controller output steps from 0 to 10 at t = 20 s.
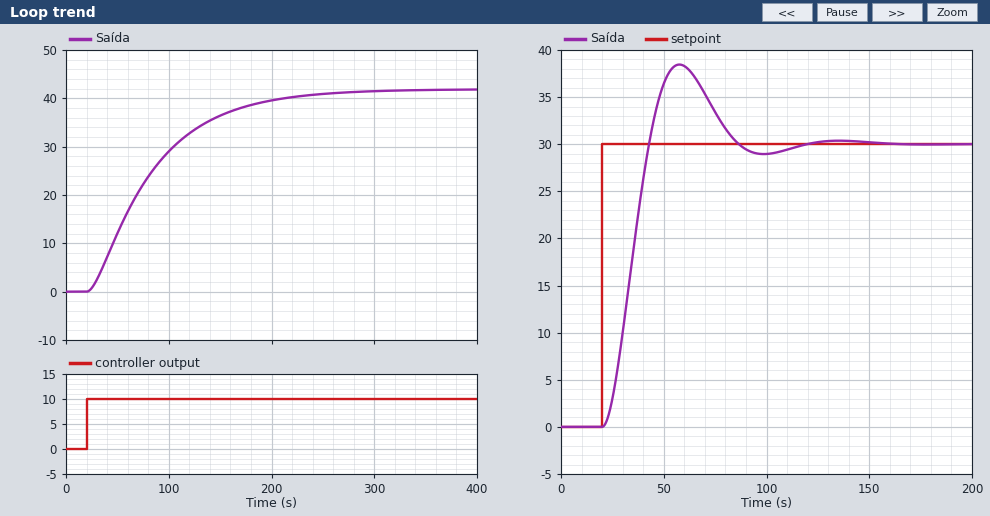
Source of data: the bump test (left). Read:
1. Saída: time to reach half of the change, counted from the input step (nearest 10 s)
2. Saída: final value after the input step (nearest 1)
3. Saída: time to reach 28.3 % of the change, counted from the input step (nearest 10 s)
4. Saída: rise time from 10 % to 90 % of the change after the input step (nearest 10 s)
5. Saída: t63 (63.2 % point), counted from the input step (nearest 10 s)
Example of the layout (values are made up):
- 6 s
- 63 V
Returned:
- 50 s
- 42
- 30 s
- 130 s
- 70 s
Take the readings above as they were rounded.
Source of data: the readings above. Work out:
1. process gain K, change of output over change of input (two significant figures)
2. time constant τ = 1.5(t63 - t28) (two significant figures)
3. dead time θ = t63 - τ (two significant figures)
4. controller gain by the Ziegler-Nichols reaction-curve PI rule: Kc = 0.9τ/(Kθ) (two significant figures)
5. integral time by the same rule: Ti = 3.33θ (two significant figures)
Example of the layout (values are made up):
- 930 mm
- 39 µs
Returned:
- 4.2
- 60 s
- 10 s
- 1.3
- 33 s
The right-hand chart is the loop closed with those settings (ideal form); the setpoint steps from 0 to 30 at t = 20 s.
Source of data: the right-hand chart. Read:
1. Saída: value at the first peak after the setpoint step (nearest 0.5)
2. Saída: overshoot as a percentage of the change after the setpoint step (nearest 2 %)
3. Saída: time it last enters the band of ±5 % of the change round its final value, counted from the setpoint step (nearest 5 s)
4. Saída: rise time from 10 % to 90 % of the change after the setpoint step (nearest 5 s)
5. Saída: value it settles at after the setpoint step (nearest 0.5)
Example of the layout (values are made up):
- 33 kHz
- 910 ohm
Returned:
- 38.5
- 28 %
- 60 s
- 15 s
- 30.0
